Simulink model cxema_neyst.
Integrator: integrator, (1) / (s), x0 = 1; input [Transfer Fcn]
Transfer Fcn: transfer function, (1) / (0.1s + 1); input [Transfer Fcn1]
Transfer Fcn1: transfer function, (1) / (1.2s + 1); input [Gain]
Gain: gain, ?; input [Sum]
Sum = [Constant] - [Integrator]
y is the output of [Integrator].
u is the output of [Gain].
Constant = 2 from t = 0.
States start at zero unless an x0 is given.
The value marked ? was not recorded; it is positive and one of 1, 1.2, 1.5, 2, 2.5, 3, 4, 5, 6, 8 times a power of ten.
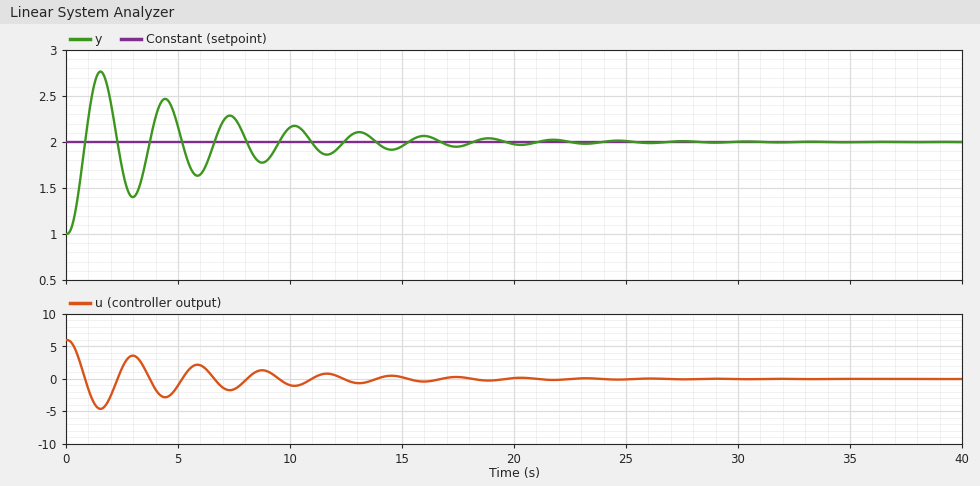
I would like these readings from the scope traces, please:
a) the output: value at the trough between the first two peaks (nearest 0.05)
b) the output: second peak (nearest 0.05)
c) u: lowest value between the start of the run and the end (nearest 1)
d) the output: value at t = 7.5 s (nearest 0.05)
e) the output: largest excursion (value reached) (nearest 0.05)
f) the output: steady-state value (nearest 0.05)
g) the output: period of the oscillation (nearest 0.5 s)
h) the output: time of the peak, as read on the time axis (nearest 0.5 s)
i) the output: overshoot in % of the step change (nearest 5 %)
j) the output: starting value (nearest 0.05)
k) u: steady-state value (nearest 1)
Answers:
1.40
2.45
-5
2.25
2.75
2.00
3.0 s
1.5 s
75 %
1.00
0
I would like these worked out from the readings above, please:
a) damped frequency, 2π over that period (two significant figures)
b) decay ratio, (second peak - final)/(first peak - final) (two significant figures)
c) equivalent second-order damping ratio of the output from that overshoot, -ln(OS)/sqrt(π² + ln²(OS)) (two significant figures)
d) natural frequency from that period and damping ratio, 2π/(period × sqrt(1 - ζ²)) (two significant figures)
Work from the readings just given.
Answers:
2.1 rad/s
0.60
0.091
2.1 rad/s
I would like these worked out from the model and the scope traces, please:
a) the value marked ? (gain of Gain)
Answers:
6
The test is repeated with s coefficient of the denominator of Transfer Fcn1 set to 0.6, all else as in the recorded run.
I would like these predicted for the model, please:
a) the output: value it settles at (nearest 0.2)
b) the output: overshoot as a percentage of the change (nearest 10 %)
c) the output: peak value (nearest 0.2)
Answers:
2.0
70 %
2.6
